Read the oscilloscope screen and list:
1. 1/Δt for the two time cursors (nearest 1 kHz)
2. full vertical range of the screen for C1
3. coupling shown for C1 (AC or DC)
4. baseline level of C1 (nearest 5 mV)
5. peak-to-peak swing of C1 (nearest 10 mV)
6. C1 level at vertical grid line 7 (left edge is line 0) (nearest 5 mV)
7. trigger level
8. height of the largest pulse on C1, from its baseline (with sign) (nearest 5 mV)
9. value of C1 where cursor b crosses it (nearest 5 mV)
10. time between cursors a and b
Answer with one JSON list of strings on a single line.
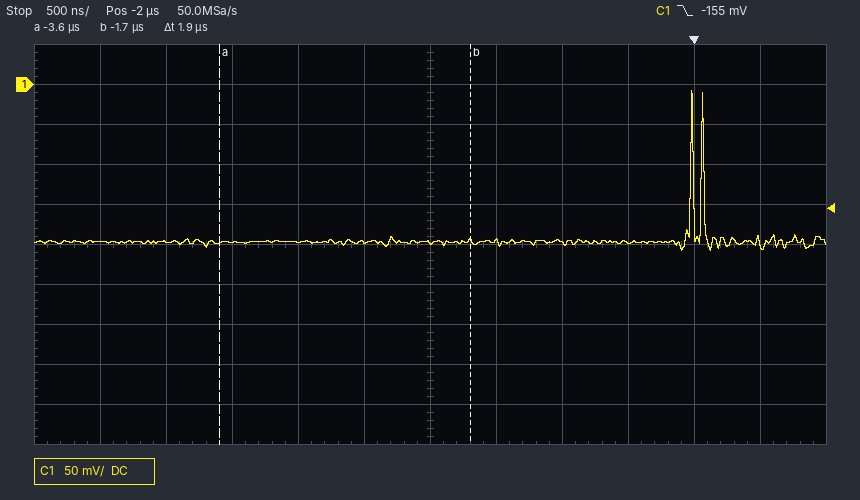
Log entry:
["526 kHz", "500 mV", "DC", "-195 mV", "200 mV", "-195 mV", "-155 mV", "+190 mV", "-195 mV", "1.9 µs"]
